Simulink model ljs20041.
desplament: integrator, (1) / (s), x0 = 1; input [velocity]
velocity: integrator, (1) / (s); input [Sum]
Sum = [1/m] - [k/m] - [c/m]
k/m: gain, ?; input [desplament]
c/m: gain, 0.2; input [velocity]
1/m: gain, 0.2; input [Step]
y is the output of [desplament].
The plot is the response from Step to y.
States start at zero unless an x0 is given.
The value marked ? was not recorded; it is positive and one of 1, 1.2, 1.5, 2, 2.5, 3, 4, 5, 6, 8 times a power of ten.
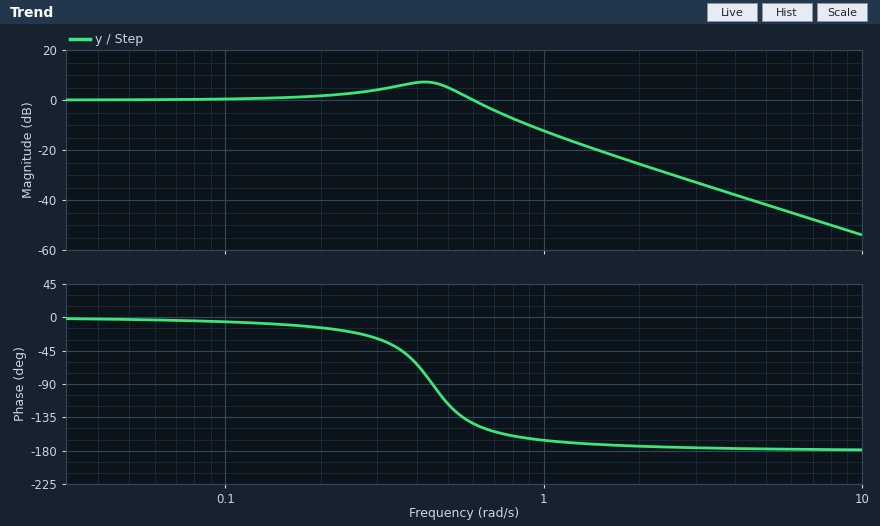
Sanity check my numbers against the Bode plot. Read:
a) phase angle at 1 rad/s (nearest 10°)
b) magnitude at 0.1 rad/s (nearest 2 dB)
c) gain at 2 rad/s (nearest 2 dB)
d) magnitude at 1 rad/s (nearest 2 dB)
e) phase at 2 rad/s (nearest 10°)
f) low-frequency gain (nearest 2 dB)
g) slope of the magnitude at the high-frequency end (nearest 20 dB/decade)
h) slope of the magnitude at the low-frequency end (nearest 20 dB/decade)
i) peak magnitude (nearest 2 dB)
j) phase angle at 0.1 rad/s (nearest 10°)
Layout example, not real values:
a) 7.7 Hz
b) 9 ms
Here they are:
a) -170°
b) 0 dB
c) -26 dB
d) -12 dB
e) -170°
f) 0 dB
g) -40 dB/decade
h) 0 dB/decade
i) 8 dB
j) -10°
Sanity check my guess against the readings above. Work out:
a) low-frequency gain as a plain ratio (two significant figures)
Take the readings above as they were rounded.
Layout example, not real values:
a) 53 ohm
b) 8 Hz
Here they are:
a) 1.0
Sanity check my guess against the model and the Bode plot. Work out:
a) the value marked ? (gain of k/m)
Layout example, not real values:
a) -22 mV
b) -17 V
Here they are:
a) 0.2
